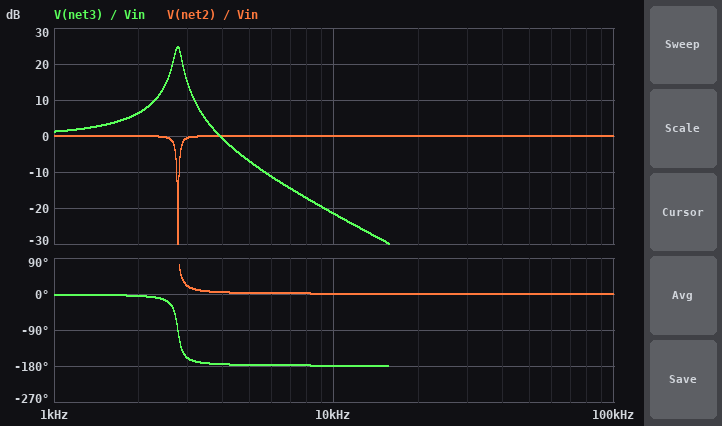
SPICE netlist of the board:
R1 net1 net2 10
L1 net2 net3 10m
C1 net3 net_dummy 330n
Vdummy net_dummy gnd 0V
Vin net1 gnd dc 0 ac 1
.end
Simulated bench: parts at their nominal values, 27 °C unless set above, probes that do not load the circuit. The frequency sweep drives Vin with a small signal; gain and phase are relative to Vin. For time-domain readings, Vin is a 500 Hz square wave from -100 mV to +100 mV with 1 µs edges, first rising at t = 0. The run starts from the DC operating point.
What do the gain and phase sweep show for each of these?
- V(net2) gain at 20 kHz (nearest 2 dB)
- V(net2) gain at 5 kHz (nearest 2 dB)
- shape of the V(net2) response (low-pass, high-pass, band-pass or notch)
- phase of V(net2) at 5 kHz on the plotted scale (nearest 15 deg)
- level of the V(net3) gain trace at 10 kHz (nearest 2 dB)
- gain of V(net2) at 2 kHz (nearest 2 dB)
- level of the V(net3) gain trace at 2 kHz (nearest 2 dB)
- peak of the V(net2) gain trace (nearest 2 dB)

0 dB
0 dB
notch
0 deg
-22 dB
0 dB
6 dB
0 dB
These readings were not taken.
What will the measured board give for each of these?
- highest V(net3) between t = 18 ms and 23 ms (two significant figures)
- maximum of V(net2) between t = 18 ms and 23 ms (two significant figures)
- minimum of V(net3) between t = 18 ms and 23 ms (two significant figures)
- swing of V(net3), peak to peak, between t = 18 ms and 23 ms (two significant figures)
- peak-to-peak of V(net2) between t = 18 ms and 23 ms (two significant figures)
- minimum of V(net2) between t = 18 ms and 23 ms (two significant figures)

250 mV
110 mV
-250 mV
500 mV
220 mV
-110 mV
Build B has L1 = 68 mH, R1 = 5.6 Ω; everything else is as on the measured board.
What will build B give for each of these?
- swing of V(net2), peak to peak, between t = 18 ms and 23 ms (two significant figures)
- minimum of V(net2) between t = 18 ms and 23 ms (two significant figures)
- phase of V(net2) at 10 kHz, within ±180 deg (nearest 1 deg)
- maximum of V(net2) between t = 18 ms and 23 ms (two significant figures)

200 mV
-100 mV
0 deg
100 mV
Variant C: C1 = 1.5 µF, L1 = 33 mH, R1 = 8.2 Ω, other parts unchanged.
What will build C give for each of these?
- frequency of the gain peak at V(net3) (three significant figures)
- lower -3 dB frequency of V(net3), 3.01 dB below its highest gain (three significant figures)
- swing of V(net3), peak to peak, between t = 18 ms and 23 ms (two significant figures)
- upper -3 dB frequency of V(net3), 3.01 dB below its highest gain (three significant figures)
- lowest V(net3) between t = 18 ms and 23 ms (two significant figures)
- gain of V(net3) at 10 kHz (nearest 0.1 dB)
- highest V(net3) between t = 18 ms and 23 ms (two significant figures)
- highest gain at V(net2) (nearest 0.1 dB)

715 Hz
695 Hz
530 mV
734 Hz
-260 mV
-45.8 dB
270 mV
0 dB
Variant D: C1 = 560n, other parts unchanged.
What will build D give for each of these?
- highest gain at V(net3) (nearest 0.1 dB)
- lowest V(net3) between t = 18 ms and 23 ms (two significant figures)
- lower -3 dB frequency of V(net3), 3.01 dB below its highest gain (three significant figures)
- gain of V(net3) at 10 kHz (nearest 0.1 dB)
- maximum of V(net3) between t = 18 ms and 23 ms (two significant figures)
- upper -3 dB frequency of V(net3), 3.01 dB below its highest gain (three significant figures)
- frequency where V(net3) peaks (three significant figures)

22.5 dB
-220 mV
2.04 kHz
-26.5 dB
220 mV
2.20 kHz
2.12 kHz
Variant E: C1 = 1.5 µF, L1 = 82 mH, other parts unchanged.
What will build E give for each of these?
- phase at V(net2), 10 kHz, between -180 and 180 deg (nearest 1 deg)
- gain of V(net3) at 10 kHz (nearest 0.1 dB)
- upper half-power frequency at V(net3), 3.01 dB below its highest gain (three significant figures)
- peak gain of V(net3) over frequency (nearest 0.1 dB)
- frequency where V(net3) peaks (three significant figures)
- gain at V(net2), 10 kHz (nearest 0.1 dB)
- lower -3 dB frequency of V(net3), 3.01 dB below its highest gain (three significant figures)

0 deg
-53.7 dB
463 Hz
27.4 dB
454 Hz
0 dB
444 Hz
